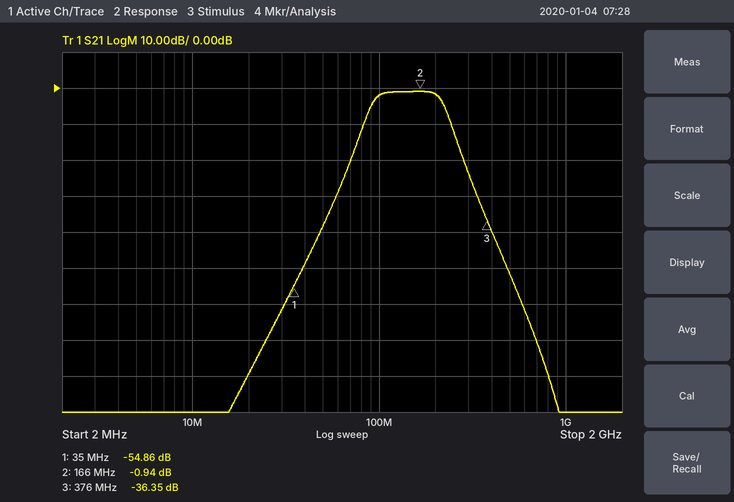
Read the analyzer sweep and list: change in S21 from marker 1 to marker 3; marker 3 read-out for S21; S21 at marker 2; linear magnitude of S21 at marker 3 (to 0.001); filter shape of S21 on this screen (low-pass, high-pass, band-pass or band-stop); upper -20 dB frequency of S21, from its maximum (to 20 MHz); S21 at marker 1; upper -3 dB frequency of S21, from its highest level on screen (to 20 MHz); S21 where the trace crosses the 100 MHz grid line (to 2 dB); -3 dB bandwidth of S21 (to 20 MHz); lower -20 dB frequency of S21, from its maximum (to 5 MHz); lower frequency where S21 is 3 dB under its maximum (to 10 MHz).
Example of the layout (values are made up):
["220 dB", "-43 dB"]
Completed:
["18.51 dB", "-36.35 dB", "-0.94 dB", "0.015", "band-pass", "280 MHz", "-54.86 dB", "220 MHz", "-2 dB", "120 MHz", "70 MHz", "90 MHz"]
